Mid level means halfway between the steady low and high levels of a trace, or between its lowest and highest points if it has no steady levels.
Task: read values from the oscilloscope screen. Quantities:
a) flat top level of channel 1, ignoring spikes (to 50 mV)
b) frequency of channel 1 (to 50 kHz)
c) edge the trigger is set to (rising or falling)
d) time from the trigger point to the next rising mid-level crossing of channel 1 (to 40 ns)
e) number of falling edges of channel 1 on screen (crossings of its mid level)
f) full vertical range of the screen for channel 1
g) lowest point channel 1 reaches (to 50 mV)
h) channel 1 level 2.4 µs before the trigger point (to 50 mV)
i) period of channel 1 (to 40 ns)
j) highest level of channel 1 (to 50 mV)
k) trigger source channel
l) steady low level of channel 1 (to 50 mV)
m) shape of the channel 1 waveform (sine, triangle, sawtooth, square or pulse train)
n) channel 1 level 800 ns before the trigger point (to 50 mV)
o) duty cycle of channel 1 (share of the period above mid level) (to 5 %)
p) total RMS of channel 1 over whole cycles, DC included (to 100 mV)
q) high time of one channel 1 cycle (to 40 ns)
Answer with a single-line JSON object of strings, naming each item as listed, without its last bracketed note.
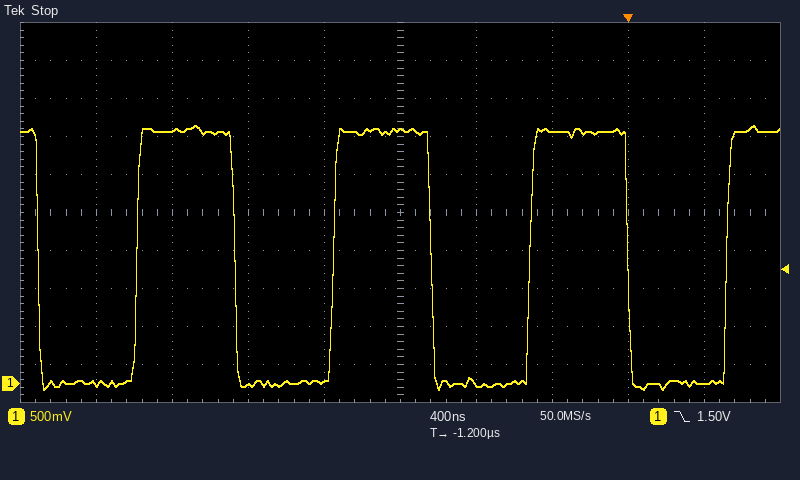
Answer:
{"flat top level of channel 1, ignoring spikes": "3.30 V", "frequency of channel 1": "950 kHz", "edge the trigger is set to": "falling", "time from the trigger point to the next rising mid-level crossing of channel 1": "520 ns", "number of falling edges of channel 1 on screen": "4", "full vertical range of the screen for channel 1": "5 V", "lowest point channel 1 reaches": "-100 mV", "channel 1 level 2.4 µs before the trigger point": "3.35 V", "period of channel 1": "1.04 µs", "highest level of channel 1": "3.40 V", "trigger source channel": "channel 1", "steady low level of channel 1": "0 mV", "shape of the channel 1 waveform": "square", "channel 1 level 800 ns before the trigger point": "0 mV", "duty cycle of channel 1 (share of the period above mid level)": "50 %", "total RMS of channel 1 over whole cycles, DC included": "2.3 V", "high time of one channel 1 cycle": "520 ns"}
